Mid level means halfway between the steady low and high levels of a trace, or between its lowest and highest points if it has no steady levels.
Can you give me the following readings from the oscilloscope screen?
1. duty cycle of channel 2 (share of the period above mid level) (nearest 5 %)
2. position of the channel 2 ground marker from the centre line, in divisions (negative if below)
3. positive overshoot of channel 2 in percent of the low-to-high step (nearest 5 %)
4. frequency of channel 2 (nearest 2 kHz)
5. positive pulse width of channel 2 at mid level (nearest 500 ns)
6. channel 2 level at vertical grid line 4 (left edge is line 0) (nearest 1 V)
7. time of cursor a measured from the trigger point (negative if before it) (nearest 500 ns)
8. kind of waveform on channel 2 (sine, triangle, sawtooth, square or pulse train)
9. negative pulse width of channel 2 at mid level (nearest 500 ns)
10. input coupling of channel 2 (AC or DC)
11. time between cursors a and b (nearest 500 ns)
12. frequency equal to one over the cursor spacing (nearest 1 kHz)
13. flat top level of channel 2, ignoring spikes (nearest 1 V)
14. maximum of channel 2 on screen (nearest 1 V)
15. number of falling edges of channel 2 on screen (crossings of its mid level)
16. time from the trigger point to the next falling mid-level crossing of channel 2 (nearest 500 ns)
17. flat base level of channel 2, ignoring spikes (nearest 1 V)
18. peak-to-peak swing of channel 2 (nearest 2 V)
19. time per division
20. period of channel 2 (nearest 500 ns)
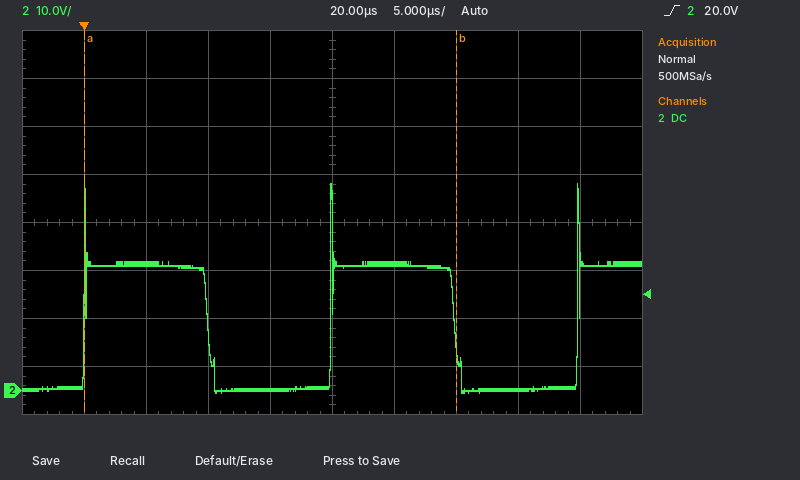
50 %
-3.5 div
65 %
50 kHz
10.0 µs
0 V
0.0 µs
square
10.0 µs
DC
30.0 µs
33 kHz
26 V
43 V
2
10.0 µs
0 V
44 V
5 µs
20.0 µs
